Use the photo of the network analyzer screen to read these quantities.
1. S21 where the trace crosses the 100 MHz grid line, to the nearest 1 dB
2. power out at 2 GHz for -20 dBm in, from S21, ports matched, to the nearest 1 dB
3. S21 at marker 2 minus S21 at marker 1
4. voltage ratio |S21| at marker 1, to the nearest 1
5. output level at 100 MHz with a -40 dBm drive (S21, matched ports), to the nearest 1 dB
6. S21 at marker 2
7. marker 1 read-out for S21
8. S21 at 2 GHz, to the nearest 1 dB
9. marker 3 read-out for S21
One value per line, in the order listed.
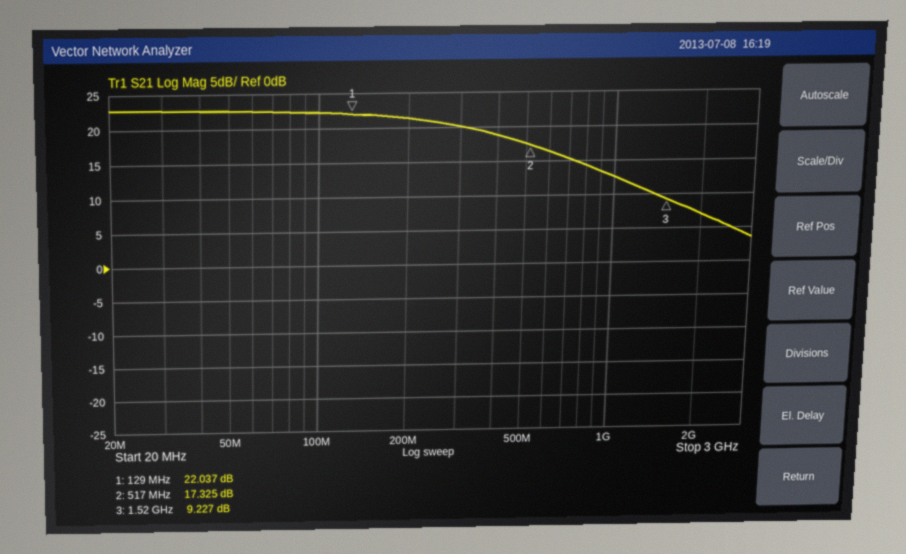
22 dB
-13 dBm
-4.712 dB
13
-18 dBm
17.325 dB
22.037 dB
7 dB
9.227 dB
